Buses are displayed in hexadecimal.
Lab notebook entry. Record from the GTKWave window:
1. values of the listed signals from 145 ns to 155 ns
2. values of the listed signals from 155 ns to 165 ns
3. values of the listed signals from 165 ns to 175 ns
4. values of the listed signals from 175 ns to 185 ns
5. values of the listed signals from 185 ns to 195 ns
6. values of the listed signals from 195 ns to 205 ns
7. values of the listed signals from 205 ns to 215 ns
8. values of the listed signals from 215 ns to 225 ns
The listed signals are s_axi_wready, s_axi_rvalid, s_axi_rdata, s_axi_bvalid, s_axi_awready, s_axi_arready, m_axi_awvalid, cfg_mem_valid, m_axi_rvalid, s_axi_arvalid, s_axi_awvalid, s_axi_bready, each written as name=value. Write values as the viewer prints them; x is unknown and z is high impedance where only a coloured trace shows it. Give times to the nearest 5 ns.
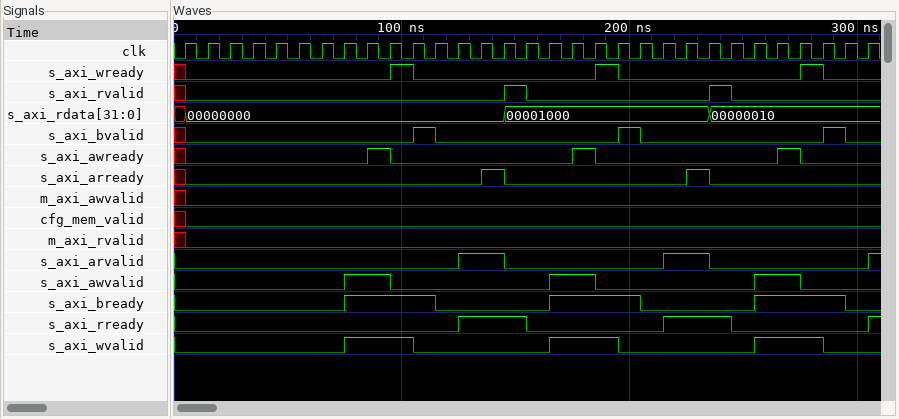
s_axi_wready=0, s_axi_rvalid=1, s_axi_rdata=00001000, s_axi_bvalid=0, s_axi_awready=0, s_axi_arready=0, m_axi_awvalid=0, cfg_mem_valid=0, m_axi_rvalid=0, s_axi_arvalid=0, s_axi_awvalid=0, s_axi_bready=0
s_axi_wready=0, s_axi_rvalid=0, s_axi_rdata=00001000, s_axi_bvalid=0, s_axi_awready=0, s_axi_arready=0, m_axi_awvalid=0, cfg_mem_valid=0, m_axi_rvalid=0, s_axi_arvalid=0, s_axi_awvalid=0, s_axi_bready=0
s_axi_wready=0, s_axi_rvalid=0, s_axi_rdata=00001000, s_axi_bvalid=0, s_axi_awready=0, s_axi_arready=0, m_axi_awvalid=0, cfg_mem_valid=0, m_axi_rvalid=0, s_axi_arvalid=0, s_axi_awvalid=1, s_axi_bready=1
s_axi_wready=0, s_axi_rvalid=0, s_axi_rdata=00001000, s_axi_bvalid=0, s_axi_awready=1, s_axi_arready=0, m_axi_awvalid=0, cfg_mem_valid=0, m_axi_rvalid=0, s_axi_arvalid=0, s_axi_awvalid=1, s_axi_bready=1
s_axi_wready=1, s_axi_rvalid=0, s_axi_rdata=00001000, s_axi_bvalid=0, s_axi_awready=0, s_axi_arready=0, m_axi_awvalid=0, cfg_mem_valid=0, m_axi_rvalid=0, s_axi_arvalid=0, s_axi_awvalid=0, s_axi_bready=1
s_axi_wready=0, s_axi_rvalid=0, s_axi_rdata=00001000, s_axi_bvalid=1, s_axi_awready=0, s_axi_arready=0, m_axi_awvalid=0, cfg_mem_valid=0, m_axi_rvalid=0, s_axi_arvalid=0, s_axi_awvalid=0, s_axi_bready=1
s_axi_wready=0, s_axi_rvalid=0, s_axi_rdata=00001000, s_axi_bvalid=0, s_axi_awready=0, s_axi_arready=0, m_axi_awvalid=0, cfg_mem_valid=0, m_axi_rvalid=0, s_axi_arvalid=0, s_axi_awvalid=0, s_axi_bready=0
s_axi_wready=0, s_axi_rvalid=0, s_axi_rdata=00001000, s_axi_bvalid=0, s_axi_awready=0, s_axi_arready=0, m_axi_awvalid=0, cfg_mem_valid=0, m_axi_rvalid=0, s_axi_arvalid=1, s_axi_awvalid=0, s_axi_bready=0
